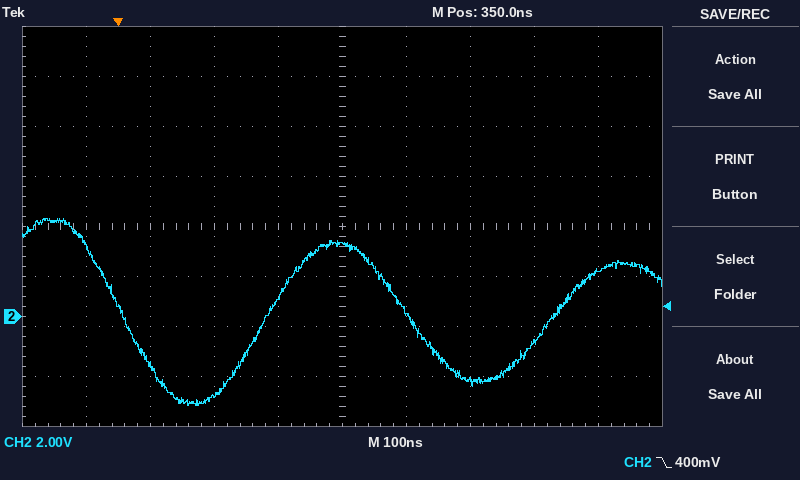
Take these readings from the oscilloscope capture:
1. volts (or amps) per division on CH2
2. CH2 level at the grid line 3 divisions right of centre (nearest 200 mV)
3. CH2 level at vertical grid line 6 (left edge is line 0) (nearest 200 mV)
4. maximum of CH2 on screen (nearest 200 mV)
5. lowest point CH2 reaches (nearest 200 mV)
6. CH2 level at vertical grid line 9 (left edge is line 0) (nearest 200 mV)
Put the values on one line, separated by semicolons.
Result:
2 V; -1.0 V; 200 mV; 4.0 V; -3.6 V; 1.8 V
